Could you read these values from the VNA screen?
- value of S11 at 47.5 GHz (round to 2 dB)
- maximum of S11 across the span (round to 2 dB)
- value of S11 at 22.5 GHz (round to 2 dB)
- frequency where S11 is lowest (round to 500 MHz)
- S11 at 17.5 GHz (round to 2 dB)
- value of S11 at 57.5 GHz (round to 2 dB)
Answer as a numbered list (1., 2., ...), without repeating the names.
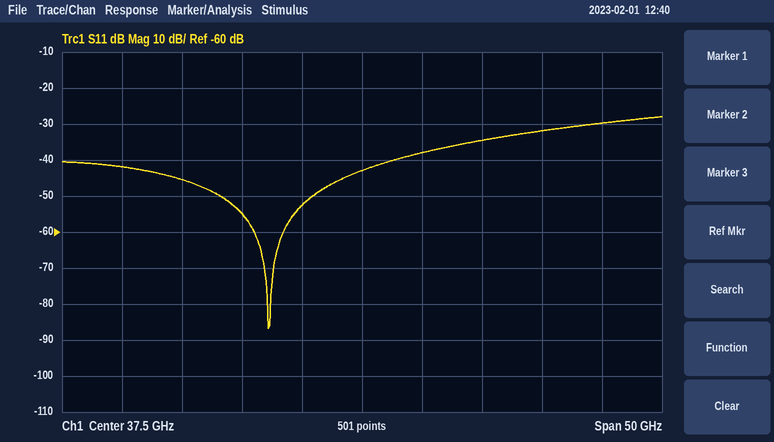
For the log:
1. -34 dB
2. -28 dB
3. -46 dB
4. 29.5 GHz
5. -42 dB
6. -30 dB
